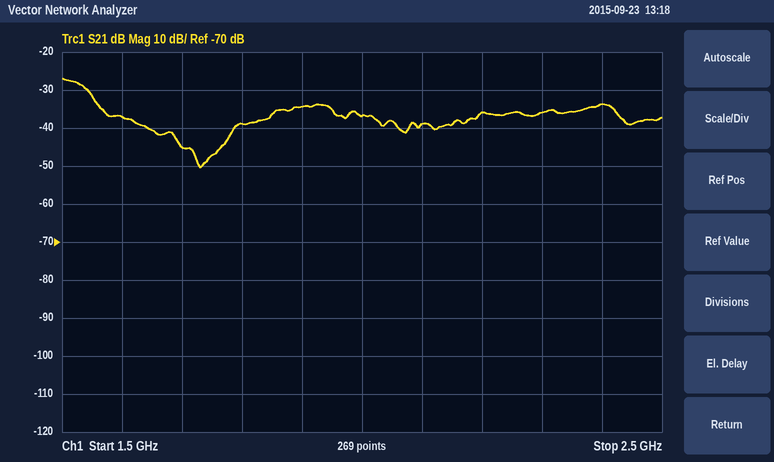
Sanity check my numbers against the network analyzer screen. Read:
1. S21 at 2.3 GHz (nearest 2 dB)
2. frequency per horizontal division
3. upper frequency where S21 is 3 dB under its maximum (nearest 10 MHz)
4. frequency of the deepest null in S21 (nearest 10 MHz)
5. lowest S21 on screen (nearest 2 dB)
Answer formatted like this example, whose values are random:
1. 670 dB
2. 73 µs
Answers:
1. -36 dB
2. 100 MHz
3. 1.54 GHz
4. 1.73 GHz
5. -50 dB
